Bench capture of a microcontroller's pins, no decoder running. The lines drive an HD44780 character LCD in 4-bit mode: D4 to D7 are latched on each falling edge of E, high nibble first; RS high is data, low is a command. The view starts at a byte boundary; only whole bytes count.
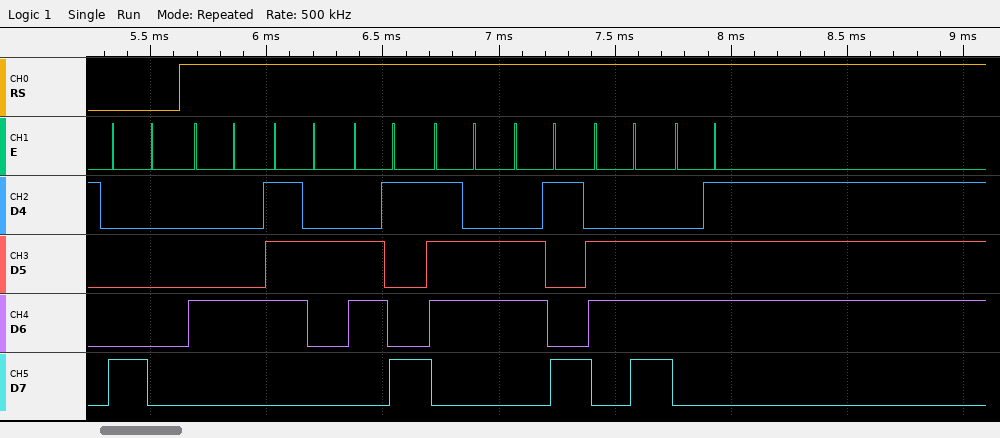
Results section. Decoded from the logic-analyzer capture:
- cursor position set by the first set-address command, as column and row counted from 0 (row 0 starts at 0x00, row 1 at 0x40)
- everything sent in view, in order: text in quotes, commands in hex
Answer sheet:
column 0, row 0
0x80 "Driving"
